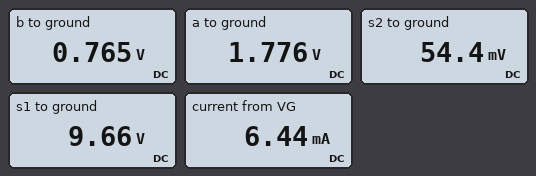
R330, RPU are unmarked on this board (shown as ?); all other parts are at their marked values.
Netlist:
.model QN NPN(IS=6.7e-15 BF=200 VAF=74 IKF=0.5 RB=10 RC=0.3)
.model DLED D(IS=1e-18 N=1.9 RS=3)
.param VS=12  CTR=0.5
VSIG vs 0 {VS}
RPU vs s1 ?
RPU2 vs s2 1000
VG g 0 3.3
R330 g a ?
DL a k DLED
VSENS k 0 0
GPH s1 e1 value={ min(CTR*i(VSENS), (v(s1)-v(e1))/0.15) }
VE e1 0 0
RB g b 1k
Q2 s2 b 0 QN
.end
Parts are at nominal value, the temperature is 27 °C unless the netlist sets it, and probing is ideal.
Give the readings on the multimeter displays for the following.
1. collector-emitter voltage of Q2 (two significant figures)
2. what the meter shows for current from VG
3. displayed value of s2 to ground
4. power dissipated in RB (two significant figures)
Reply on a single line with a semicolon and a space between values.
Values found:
54 mV; 6.44 mA; 54.4 mV; 6.4 mW
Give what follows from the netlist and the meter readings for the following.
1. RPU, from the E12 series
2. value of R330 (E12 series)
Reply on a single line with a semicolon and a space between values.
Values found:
1.2 kΩ; 390 Ω
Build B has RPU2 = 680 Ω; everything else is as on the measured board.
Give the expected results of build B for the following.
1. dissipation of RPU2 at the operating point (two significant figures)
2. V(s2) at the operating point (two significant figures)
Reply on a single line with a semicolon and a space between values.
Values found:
210 mW; 64 mV
